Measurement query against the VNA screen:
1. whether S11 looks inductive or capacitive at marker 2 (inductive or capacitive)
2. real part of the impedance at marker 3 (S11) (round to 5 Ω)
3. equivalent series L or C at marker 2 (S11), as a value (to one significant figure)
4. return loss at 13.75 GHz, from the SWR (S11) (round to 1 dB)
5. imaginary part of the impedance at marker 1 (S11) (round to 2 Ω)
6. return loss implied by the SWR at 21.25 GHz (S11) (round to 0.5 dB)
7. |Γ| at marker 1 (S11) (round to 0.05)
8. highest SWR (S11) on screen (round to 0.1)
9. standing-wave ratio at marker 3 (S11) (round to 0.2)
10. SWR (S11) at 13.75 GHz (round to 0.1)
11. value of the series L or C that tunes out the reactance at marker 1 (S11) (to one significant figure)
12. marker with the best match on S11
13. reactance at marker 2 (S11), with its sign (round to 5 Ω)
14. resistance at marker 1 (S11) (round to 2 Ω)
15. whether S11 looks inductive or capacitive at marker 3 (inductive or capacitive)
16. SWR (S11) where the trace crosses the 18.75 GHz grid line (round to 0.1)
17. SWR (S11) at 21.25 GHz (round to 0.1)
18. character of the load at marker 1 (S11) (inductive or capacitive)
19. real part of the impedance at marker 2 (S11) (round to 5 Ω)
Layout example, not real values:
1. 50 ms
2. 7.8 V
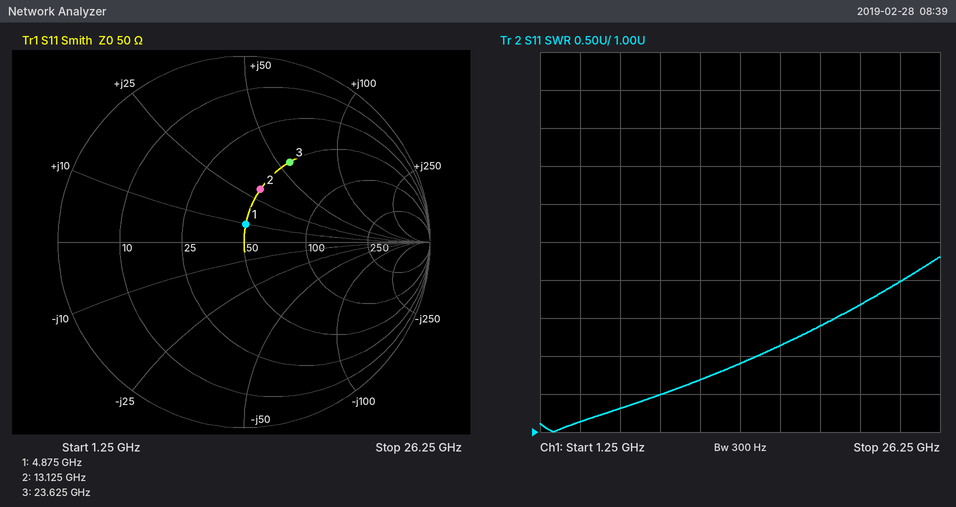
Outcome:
1. inductive
2. 50 Ω
3. 400 pH
4. 10 dB
5. +10 Ω
6. 7.0 dB
7. 0.10
8. 3.3
9. 3.0
10. 1.9
11. 3 pF
12. marker 1
13. +30 Ω
14. 50 Ω
15. inductive
16. 2.4
17. 2.7
18. inductive
19. 50 Ω
